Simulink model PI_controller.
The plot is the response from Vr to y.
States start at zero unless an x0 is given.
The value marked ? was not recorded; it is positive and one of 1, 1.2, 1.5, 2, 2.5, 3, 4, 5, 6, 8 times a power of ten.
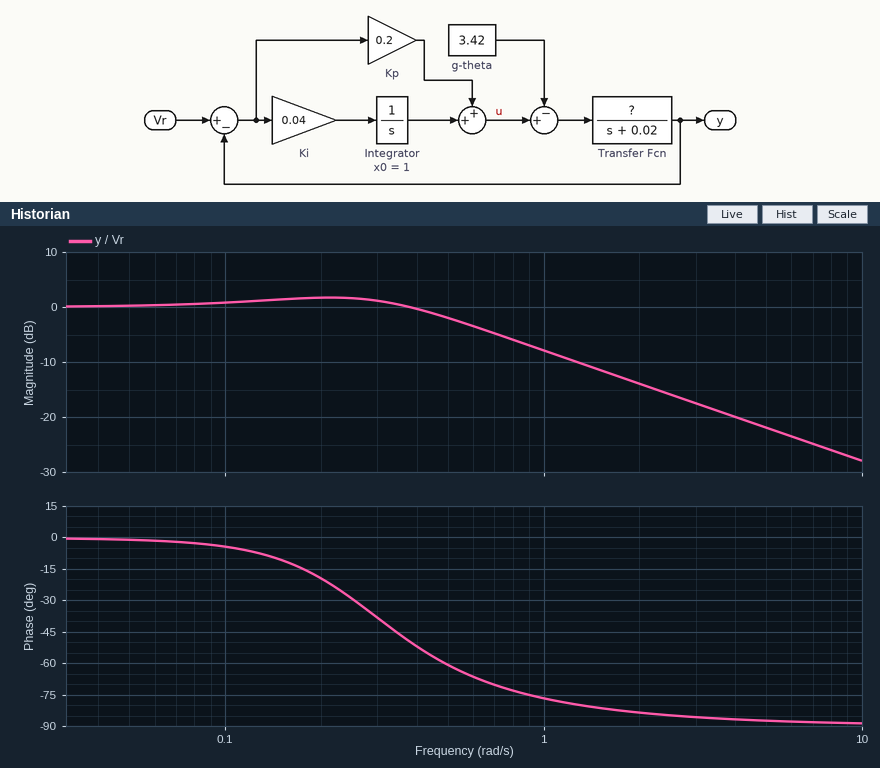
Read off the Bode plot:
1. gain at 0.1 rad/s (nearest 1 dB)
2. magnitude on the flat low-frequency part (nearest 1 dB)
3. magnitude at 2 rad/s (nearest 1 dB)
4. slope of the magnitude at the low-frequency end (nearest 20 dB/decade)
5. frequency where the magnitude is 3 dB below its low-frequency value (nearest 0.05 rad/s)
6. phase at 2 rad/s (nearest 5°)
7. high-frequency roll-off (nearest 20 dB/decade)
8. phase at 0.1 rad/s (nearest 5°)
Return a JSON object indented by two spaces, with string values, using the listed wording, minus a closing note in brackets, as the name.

{
  "gain at 0.1 rad/s": "1 dB",
  "magnitude on the flat low-frequency part": "0 dB",
  "magnitude at 2 rad/s": "-14 dB",
  "slope of the magnitude at the low-frequency end": "0 dB/decade",
  "frequency where the magnitude is 3 dB below its low-frequency value": "0.55 rad/s",
  "phase at 2 rad/s": "-85°",
  "high-frequency roll-off": "-20 dB/decade",
  "phase at 0.1 rad/s": "-5°"
}
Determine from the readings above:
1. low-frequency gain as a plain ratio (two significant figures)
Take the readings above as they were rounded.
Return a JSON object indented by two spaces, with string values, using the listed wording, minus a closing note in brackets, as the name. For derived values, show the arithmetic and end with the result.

{
  "low-frequency gain as a plain ratio": "10^(0 / 20) = 1.0"
}
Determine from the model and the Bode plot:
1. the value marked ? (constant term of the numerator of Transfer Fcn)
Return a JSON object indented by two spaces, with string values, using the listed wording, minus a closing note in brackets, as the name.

{
  "the value marked ?": "2"
}
